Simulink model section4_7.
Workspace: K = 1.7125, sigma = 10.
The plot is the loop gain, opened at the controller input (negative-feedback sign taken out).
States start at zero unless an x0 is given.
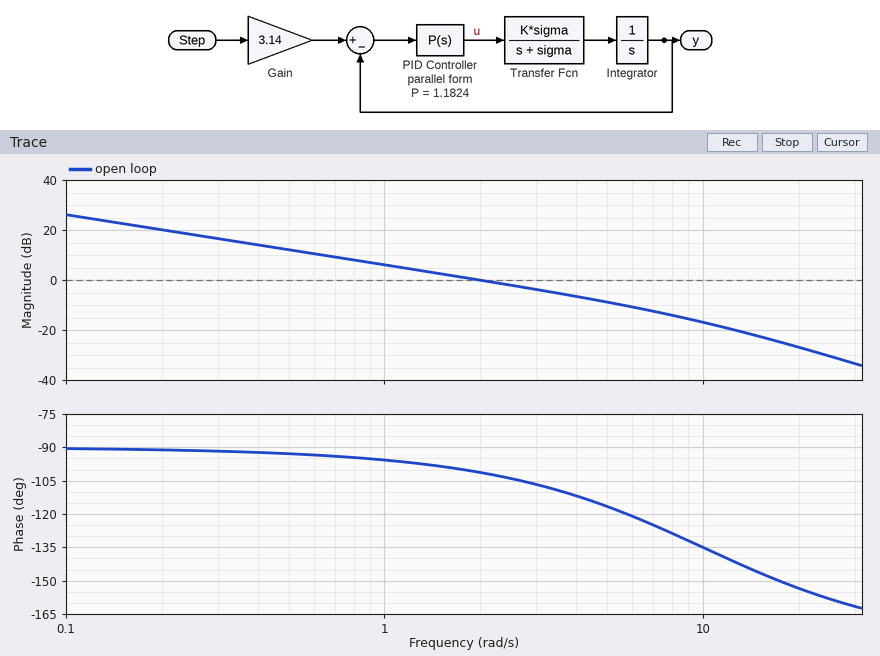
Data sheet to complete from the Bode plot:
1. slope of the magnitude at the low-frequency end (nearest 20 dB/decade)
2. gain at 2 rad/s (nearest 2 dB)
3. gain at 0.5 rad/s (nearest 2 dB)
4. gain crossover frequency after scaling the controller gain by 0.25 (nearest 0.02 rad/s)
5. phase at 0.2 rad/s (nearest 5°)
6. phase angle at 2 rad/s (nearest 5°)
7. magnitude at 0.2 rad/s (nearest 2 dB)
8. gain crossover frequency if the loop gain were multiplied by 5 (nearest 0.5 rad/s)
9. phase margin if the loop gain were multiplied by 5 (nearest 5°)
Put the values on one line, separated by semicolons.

-20 dB/decade; 0 dB; 12 dB; 0.50 rad/s; -90°; -100°; 20 dB; 8.0 rad/s; 50°
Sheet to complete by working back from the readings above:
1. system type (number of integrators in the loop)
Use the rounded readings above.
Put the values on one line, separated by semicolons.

1
